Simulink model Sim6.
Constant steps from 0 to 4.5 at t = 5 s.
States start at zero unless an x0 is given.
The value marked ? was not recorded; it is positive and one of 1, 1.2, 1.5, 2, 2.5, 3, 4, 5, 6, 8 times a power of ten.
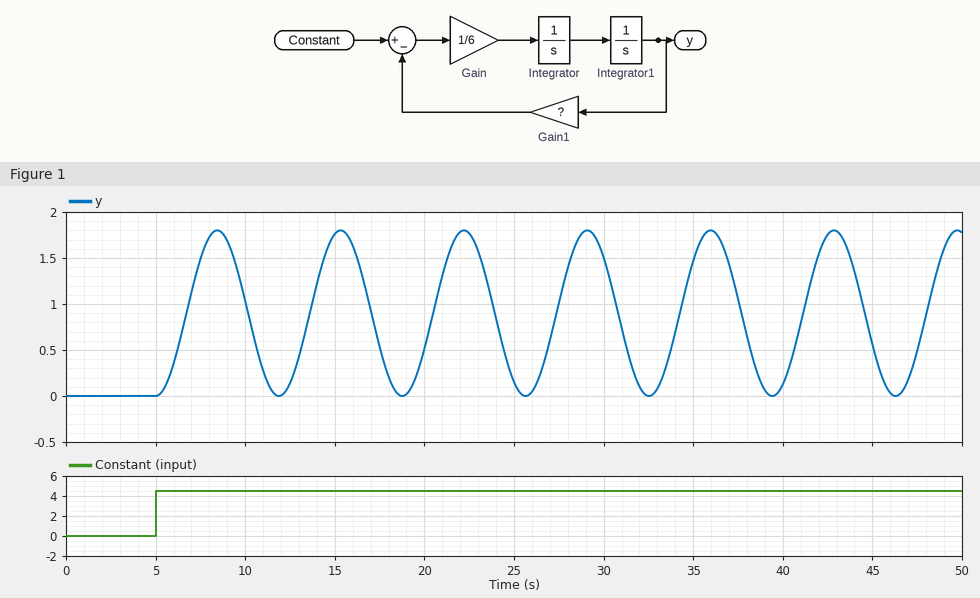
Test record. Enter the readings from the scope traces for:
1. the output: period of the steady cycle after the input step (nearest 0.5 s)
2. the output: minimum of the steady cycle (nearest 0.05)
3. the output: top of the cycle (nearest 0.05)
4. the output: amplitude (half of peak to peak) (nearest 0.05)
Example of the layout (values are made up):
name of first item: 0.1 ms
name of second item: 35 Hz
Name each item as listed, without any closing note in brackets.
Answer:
the output: period of the steady cycle after the input step: 7.0 s
the output: minimum of the steady cycle: 0.00
the output: top of the cycle: 1.80
the output: amplitude (half of peak to peak): 0.90
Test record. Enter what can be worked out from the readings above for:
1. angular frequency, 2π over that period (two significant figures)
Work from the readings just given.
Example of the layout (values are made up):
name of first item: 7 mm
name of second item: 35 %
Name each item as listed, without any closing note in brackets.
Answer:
angular frequency, 2π over that period: 0.90 rad/s
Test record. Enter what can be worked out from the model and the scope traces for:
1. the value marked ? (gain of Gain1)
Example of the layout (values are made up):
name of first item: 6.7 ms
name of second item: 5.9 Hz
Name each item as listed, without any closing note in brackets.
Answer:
the value marked ?: 5
